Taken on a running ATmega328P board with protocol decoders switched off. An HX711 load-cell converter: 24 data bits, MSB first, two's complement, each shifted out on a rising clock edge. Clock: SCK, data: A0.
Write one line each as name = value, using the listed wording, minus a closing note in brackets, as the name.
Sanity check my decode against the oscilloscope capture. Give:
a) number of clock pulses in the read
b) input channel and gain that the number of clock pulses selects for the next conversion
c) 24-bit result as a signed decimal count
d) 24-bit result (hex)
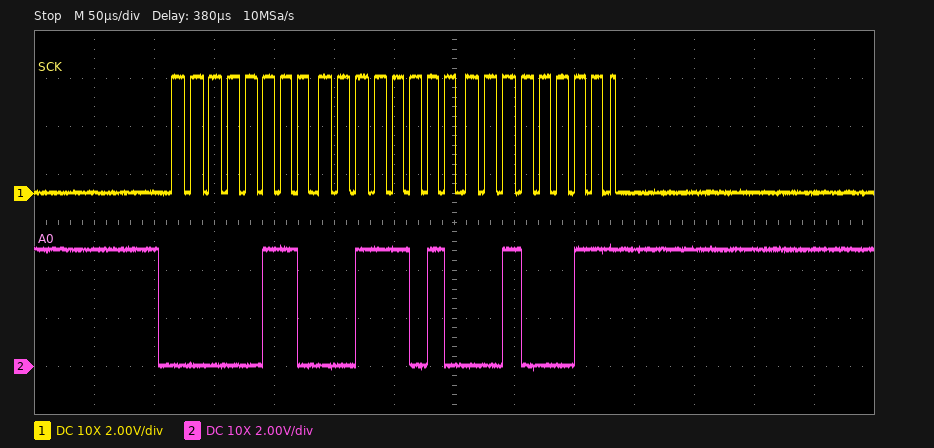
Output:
number of clock pulses in the read = 25
input channel and gain that the number of clock pulses selects for the next conversion = channel A, gain 128
24-bit result as a signed decimal count = 408099
24-bit result = 0x063A23
